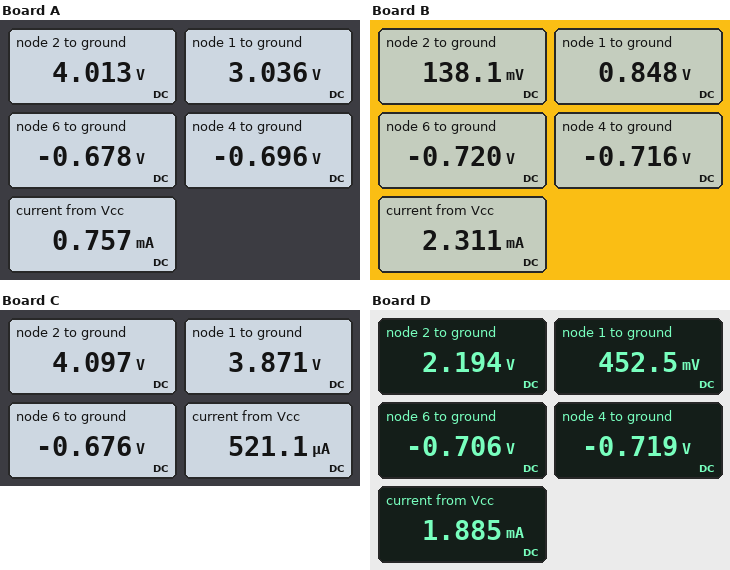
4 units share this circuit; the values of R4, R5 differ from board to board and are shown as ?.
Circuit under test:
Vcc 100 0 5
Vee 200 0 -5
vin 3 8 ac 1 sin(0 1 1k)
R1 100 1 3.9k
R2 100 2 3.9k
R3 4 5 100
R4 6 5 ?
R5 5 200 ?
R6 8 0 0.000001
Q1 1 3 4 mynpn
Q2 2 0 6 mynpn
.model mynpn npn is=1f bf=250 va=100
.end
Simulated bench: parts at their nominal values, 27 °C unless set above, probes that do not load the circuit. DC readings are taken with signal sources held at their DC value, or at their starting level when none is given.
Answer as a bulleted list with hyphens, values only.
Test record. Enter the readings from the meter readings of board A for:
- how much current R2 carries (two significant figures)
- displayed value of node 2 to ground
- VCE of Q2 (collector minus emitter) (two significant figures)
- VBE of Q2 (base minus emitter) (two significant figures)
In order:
- 250 µA
- 4.013 V
- 4.7 V
- 680 mV
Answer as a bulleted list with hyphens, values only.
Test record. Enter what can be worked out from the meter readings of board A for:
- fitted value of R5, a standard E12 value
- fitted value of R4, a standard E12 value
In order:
- 5.6 kΩ
- 270 Ω
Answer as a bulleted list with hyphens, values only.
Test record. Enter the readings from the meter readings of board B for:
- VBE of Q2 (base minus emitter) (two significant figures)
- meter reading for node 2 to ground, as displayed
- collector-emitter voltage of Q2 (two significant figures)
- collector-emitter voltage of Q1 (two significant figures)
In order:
- 720 mV
- 138.1 mV
- 860 mV
- 1.6 V
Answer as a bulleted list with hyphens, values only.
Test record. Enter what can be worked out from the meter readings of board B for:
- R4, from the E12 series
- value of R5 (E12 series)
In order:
- 82 Ω
- 1.8 kΩ
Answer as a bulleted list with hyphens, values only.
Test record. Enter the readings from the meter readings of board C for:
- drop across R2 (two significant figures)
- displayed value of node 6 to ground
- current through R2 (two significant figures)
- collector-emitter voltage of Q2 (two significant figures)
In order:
- 900 mV
- -0.676 V
- 230 µA
- 4.8 V
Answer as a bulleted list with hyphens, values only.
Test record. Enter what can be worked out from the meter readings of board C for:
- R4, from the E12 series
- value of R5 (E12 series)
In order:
- 150 Ω
- 8.2 kΩ
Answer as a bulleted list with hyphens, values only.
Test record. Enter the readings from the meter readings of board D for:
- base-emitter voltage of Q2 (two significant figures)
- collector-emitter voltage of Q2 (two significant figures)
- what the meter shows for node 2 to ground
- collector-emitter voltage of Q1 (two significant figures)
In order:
- 710 mV
- 2.9 V
- 2.194 V
- 1.2 V
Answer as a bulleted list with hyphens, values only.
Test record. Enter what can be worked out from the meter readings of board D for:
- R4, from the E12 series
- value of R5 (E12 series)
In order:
- 180 Ω
- 2.2 kΩ
